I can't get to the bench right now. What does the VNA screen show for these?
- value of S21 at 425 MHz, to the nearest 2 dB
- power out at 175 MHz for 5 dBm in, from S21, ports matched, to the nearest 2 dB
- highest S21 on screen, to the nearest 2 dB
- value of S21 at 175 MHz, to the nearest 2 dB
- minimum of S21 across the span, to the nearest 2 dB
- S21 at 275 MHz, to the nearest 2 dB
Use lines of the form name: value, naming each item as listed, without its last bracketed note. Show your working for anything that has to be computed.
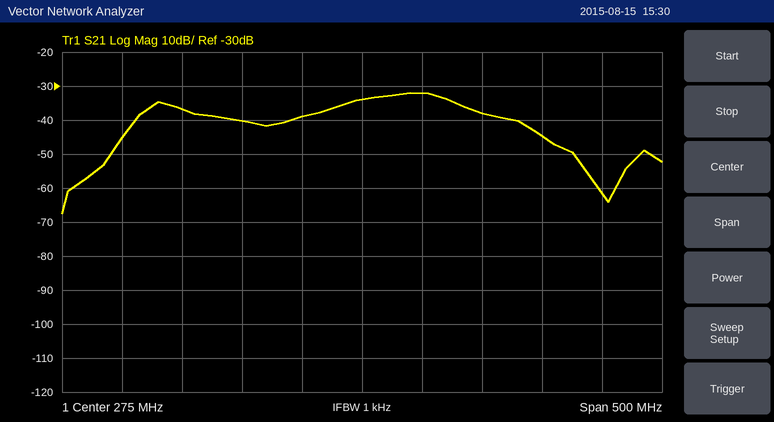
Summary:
value of S21 at 425 MHz, to the nearest 2 dB: -44 dB
power out at 175 MHz for 5 dBm in, from S21, ports matched, to the nearest 2 dB: 5 dBm + (-40 dB) = -36 dBm
highest S21 on screen, to the nearest 2 dB: -32 dB
value of S21 at 175 MHz, to the nearest 2 dB: -40 dB
minimum of S21 across the span, to the nearest 2 dB: -68 dB
S21 at 275 MHz, to the nearest 2 dB: -34 dB
